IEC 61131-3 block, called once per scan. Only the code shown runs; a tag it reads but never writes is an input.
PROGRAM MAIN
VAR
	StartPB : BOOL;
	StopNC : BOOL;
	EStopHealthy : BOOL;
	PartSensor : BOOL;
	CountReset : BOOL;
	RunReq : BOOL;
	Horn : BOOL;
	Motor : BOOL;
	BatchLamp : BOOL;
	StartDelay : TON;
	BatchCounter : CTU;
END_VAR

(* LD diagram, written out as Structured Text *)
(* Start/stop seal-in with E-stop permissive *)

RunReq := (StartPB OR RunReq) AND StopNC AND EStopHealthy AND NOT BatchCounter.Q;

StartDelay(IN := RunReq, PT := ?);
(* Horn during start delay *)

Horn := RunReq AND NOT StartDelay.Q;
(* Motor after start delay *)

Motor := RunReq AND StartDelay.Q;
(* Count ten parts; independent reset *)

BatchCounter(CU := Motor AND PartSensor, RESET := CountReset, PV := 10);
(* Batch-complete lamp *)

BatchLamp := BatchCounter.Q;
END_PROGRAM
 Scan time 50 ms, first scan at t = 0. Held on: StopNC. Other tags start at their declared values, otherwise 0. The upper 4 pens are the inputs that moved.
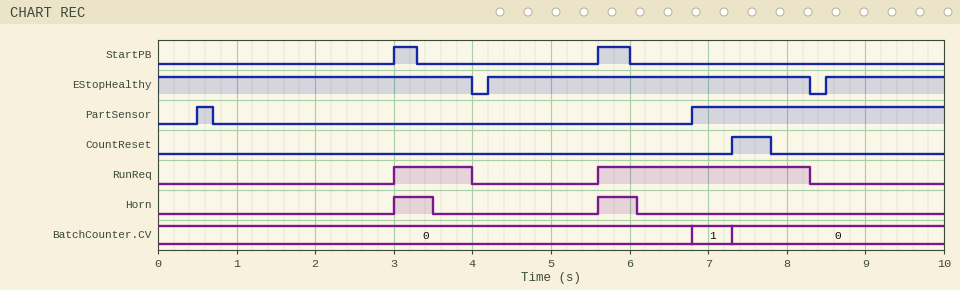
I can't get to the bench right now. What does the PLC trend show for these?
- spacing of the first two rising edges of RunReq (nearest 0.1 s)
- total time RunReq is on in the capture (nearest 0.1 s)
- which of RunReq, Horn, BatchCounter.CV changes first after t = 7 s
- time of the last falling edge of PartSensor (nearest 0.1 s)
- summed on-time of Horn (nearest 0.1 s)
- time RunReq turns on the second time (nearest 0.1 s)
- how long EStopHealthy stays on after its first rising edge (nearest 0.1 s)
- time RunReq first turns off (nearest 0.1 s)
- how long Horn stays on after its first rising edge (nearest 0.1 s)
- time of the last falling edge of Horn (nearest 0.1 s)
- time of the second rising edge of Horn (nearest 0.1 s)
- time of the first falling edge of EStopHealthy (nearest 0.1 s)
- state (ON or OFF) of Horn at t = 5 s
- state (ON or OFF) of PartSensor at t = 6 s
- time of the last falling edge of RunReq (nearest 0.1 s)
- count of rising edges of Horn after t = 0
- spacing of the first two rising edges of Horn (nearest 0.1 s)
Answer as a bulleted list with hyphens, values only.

- 2.6 s
- 3.7 s
- BatchCounter.CV
- 0.7 s
- 1.0 s
- 5.6 s
- 4.1 s
- 4.0 s
- 0.5 s
- 6.1 s
- 5.6 s
- 4.0 s
- OFF
- OFF
- 8.3 s
- 2
- 2.6 s
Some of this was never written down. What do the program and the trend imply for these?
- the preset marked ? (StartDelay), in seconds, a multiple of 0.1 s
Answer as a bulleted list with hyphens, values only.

- 0.5 s
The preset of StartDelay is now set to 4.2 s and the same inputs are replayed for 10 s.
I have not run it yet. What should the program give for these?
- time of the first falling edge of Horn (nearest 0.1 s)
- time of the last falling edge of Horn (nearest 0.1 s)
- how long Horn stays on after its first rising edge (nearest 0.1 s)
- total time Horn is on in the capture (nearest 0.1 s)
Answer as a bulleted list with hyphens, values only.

- 4.0 s
- 8.3 s
- 1.0 s
- 3.7 s
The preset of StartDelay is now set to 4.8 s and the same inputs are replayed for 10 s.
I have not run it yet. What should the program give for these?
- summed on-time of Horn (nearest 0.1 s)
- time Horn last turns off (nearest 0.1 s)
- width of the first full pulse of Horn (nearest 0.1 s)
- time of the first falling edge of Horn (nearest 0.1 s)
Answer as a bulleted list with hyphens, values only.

- 3.7 s
- 8.3 s
- 1.0 s
- 4.0 s
